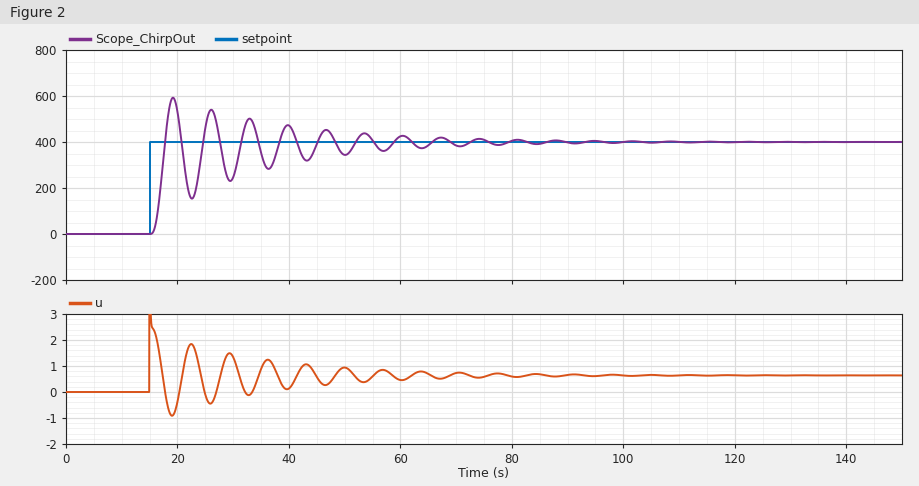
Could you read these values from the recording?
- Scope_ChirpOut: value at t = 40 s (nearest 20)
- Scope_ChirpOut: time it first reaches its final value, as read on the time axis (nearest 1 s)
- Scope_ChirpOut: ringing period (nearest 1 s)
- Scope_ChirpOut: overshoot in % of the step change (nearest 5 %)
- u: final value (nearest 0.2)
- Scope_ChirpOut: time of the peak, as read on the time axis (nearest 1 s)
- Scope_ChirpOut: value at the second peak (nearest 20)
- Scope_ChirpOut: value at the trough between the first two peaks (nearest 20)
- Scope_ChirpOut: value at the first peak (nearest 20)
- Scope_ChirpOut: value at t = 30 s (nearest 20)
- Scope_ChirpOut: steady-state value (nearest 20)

480
18 s
7 s
50 %
0.6
19 s
540
160
600
240
400
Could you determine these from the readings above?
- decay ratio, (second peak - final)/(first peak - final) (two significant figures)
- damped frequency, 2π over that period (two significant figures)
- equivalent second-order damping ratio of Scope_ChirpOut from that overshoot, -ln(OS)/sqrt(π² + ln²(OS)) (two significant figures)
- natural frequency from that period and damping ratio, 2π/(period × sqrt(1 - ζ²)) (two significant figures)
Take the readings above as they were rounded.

0.70
0.90 rad/s
0.22
0.92 rad/s
